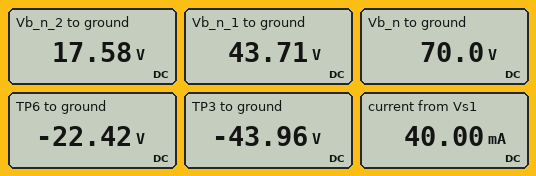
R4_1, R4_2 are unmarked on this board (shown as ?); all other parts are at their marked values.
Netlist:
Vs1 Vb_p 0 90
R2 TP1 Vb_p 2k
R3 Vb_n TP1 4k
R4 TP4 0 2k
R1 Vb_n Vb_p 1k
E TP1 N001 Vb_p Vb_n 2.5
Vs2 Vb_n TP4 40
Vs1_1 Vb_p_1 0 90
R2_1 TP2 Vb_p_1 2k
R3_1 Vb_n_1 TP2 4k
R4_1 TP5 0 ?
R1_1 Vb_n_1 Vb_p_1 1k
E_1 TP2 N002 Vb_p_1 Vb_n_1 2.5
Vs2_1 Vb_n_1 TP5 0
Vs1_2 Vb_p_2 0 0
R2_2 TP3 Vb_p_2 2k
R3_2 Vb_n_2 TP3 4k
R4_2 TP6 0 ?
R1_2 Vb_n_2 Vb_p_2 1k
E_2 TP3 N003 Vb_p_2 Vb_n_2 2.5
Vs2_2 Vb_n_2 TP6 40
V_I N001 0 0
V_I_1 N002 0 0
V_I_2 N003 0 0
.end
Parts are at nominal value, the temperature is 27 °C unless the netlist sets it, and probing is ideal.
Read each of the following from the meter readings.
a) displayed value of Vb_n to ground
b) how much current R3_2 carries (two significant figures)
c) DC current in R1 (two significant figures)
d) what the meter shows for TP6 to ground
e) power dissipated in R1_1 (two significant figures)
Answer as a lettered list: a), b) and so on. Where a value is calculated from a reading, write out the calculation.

a) 70.0 V
b) (17.58 V - (-43.96 V)) / 4 kΩ = 15 mA
c) (90 V - 70 V) / 1 kΩ = 20 mA
d) -22.42 V
e) (90 V - 43.71 V)^2 / 1 kΩ = 2.1 W
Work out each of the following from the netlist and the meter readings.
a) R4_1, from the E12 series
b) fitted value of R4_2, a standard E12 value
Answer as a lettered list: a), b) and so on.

a) 680 Ω
b) 680 Ω
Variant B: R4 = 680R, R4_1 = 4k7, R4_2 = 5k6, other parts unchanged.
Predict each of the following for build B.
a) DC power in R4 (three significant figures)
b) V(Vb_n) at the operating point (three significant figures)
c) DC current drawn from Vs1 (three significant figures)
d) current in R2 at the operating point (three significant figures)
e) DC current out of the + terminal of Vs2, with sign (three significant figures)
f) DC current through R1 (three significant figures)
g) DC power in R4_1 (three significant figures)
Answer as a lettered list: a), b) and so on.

a) 667 mW
b) 61.3 V
c) 37.8 mA
d) 9.12 mA
e) -31.3 mA
f) 28.7 mA
g) 1.04 W
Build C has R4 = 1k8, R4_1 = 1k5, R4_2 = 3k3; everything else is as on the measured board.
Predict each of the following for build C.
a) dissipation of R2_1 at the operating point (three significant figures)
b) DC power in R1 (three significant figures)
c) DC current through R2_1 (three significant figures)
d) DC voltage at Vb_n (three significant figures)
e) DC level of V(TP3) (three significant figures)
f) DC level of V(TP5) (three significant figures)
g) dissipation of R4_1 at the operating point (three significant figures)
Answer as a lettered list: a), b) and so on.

a) 39.2 mW
b) 428 mW
c) 4.43 mA
d) 69.3 V
e) -13.9 V
f) 57.5 V
g) 2.21 W
